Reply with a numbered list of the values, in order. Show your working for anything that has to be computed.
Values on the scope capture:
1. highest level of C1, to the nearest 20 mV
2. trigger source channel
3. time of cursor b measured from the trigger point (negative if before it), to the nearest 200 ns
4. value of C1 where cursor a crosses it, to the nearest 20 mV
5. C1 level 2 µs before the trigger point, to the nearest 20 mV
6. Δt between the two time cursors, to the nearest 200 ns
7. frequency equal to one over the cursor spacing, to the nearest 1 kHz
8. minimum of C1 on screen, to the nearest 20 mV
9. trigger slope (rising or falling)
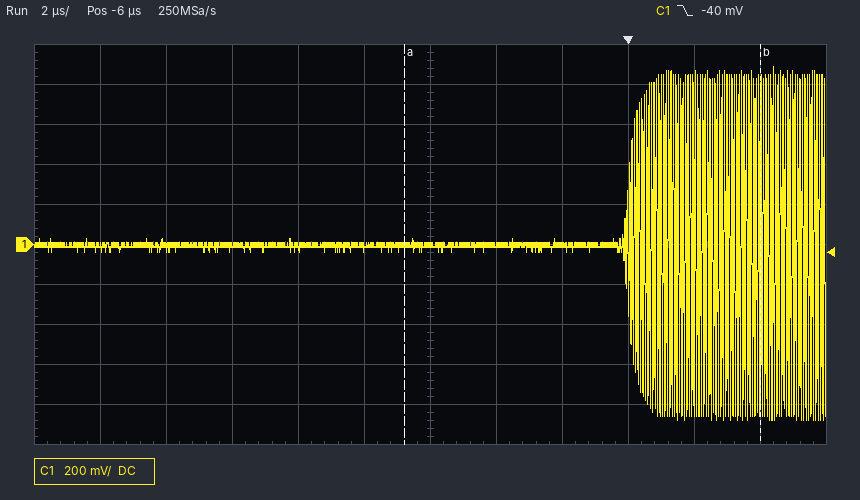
1. 900 mV
2. C1
3. +4.0 µs
4. 0 mV
5. 0 mV
6. 10.8 µs
7. 1 / 10.8 µs ≈ 93 kHz
8. -880 mV
9. falling
